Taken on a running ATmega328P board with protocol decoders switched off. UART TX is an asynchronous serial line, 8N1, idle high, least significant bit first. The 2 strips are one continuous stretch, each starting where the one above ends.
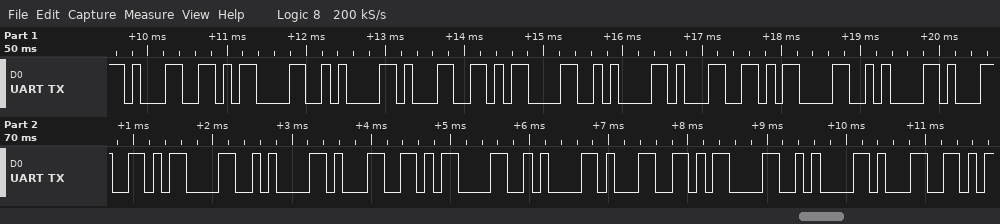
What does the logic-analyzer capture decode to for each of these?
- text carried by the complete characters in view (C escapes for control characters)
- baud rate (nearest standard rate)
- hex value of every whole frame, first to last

"1\r\n1\r\n1\r\n1\r\n1\r\n1\r\n1"
9600 baud
0x31 0x0D 0x0A 0x31 0x0D 0x0A 0x31 0x0D 0x0A 0x31 0x0D 0x0A 0x31 0x0D 0x0A 0x31 0x0D 0x0A 0x31
